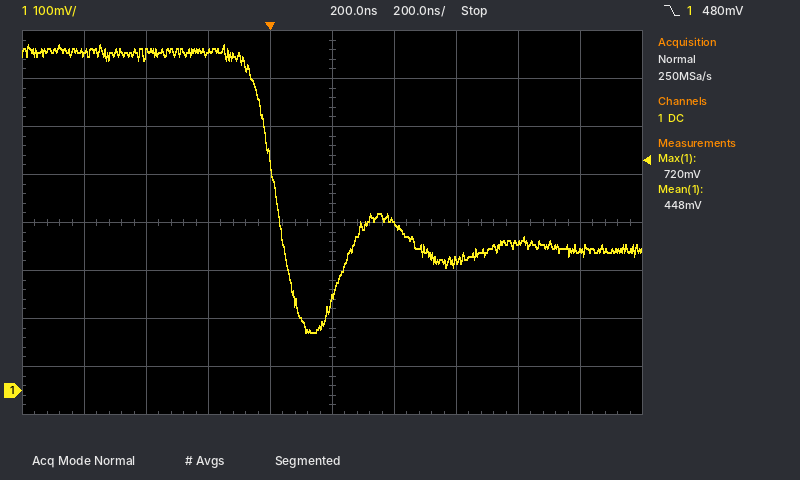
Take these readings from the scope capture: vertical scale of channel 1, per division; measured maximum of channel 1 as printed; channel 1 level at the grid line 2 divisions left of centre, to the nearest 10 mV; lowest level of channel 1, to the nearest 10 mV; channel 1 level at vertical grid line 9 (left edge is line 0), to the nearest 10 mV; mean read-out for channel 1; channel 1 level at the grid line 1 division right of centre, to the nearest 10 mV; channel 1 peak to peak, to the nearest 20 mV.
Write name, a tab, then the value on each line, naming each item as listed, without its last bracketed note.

vertical scale of channel 1, per division	100 mV
measured maximum of channel 1 as printed	720 mV
channel 1 level at the grid line 2 divisions left of centre, to the nearest 10 mV	700 mV
lowest level of channel 1, to the nearest 10 mV	120 mV
channel 1 level at vertical grid line 9 (left edge is line 0), to the nearest 10 mV	290 mV
mean read-out for channel 1	448 mV
channel 1 level at the grid line 1 division right of centre, to the nearest 10 mV	350 mV
channel 1 peak to peak, to the nearest 20 mV	600 mV
